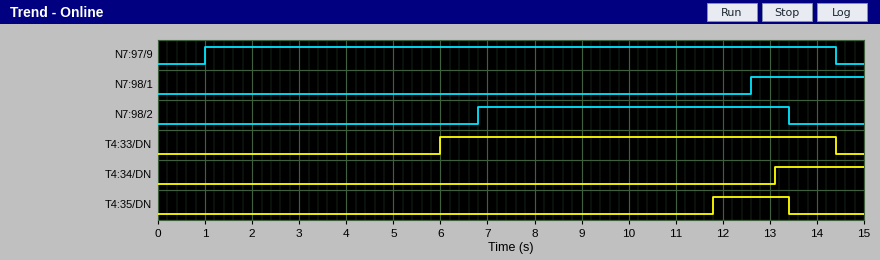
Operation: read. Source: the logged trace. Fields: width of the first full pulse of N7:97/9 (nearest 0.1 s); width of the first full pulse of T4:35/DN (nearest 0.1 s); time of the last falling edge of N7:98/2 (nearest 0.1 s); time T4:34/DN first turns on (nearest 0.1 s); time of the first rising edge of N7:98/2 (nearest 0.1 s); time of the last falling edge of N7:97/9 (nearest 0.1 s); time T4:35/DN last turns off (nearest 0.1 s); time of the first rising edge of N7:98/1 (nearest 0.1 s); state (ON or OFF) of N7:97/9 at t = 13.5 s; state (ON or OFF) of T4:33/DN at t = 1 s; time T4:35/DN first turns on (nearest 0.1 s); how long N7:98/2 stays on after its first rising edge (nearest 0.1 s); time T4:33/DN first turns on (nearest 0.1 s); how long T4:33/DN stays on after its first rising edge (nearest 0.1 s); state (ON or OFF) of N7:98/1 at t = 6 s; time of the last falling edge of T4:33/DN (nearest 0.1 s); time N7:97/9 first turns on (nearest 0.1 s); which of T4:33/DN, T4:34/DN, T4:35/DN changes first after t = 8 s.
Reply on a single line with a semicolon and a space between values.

13.4 s; 1.6 s; 13.4 s; 13.1 s; 6.8 s; 14.4 s; 13.4 s; 12.6 s; ON; OFF; 11.8 s; 6.6 s; 6.0 s; 8.4 s; OFF; 14.4 s; 1.0 s; T4:35/DN
